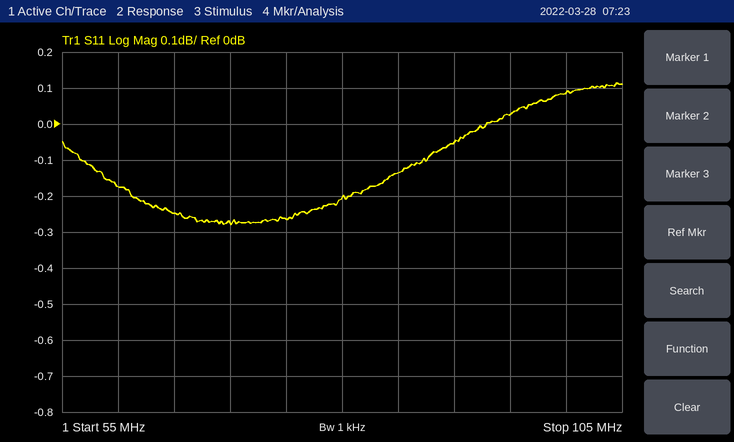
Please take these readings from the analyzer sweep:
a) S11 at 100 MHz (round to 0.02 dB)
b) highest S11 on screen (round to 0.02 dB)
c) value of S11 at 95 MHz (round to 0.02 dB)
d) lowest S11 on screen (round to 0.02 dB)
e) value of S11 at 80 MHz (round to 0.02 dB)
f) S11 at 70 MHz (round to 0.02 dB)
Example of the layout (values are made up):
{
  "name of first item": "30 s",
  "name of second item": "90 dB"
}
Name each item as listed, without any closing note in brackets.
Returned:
{
  "S11 at 100 MHz": "0.08 dB",
  "highest S11 on screen": "0.12 dB",
  "value of S11 at 95 MHz": "0.02 dB",
  "lowest S11 on screen": "-0.28 dB",
  "value of S11 at 80 MHz": "-0.20 dB",
  "S11 at 70 MHz": "-0.28 dB"
}
